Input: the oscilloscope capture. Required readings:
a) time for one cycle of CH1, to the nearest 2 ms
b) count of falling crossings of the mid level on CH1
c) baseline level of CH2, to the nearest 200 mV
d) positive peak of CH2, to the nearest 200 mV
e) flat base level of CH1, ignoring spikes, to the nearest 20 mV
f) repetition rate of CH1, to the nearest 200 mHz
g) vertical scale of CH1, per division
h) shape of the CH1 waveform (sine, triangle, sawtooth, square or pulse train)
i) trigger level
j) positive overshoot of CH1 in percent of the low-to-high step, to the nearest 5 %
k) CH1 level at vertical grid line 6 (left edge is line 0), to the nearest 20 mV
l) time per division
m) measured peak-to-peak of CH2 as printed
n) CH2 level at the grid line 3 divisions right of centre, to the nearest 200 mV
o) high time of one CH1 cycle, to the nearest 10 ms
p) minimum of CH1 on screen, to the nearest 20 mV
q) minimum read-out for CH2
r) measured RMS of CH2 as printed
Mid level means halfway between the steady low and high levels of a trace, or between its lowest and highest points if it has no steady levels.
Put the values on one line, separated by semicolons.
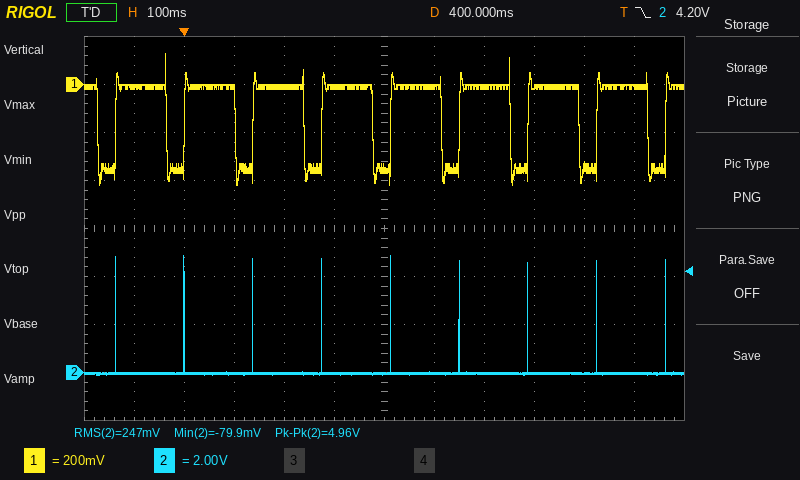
138 ms; 9; 0.0 V; 4.8 V; -360 mV; 7.2 Hz; 200 mV; pulse train; 4.20 V; 40 %; -340 mV; 100 ms; 4.96 V; 0.0 V; 100 ms; -420 mV; -79.9 mV; 247 mV
